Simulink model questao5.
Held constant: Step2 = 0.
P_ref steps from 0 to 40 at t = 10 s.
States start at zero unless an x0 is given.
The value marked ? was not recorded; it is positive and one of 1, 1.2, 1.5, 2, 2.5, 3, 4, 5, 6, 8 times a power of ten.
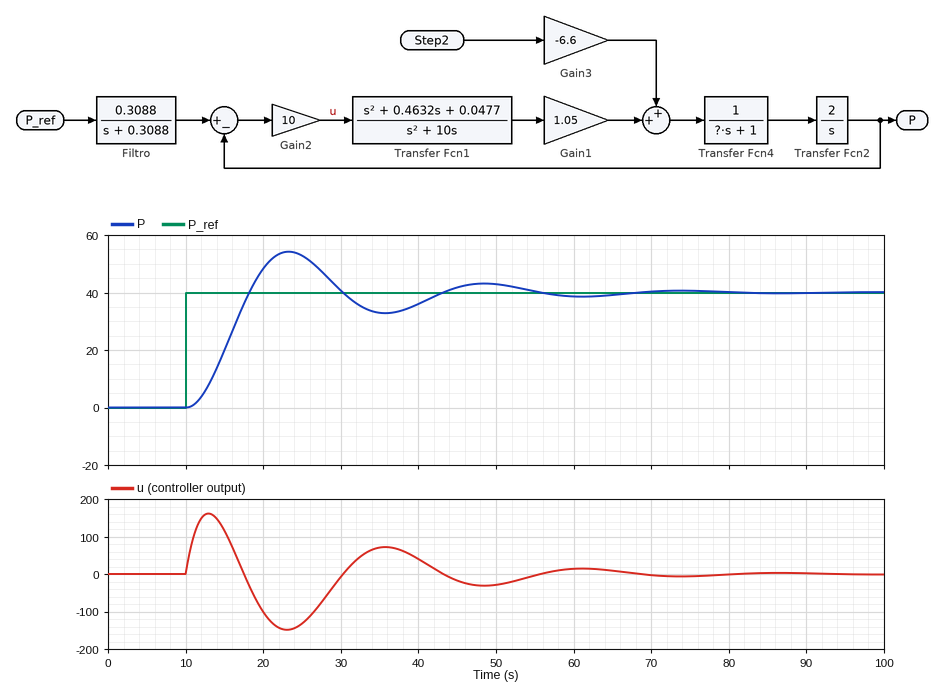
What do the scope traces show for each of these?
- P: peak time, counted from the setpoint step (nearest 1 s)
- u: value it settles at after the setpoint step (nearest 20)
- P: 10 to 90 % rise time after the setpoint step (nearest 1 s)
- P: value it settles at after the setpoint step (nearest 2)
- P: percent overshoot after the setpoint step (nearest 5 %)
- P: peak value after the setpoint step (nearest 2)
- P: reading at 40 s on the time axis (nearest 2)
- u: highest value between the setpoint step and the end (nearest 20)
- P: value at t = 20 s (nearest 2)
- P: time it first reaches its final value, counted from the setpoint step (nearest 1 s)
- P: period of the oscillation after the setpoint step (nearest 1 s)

13 s
0
5 s
40
35 %
54
36
160
48
8 s
25 s
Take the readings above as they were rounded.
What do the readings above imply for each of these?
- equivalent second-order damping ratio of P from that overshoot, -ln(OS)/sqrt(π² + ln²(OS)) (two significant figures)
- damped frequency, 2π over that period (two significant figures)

0.32
0.25 rad/s
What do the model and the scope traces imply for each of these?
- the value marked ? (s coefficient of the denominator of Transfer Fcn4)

12
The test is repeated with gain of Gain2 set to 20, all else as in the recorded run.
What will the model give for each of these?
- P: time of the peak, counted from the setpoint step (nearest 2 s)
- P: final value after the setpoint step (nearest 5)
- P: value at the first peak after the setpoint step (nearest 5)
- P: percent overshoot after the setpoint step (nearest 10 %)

10 s
40
45
20 %
